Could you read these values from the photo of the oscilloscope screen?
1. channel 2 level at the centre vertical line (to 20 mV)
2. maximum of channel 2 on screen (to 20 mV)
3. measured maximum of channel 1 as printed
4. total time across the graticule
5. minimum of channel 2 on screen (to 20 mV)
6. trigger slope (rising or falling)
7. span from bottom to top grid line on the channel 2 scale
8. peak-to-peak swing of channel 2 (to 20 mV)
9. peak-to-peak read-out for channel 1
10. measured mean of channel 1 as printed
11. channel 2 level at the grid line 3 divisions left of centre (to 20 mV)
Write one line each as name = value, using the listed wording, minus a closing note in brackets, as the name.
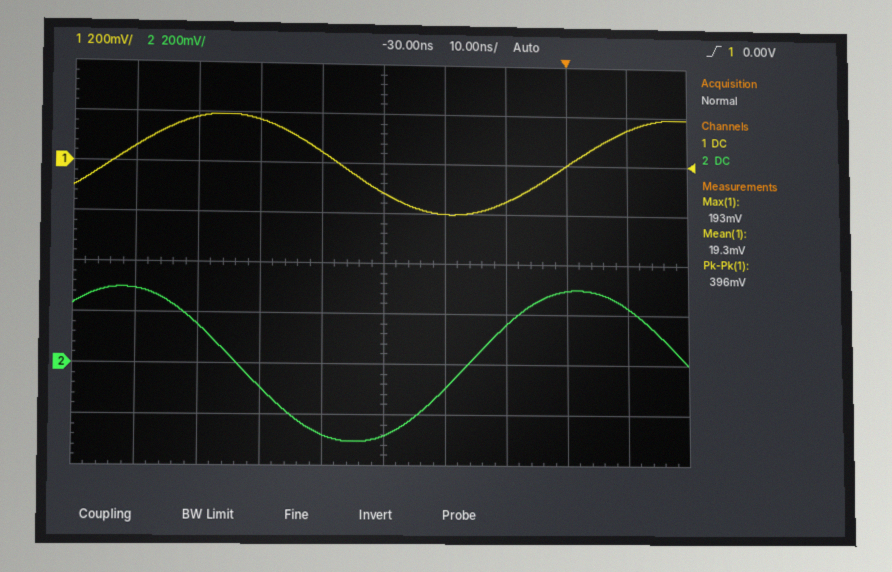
channel 2 level at the centre vertical line = -280 mV
maximum of channel 2 on screen = 300 mV
measured maximum of channel 1 as printed = 193 mV
total time across the graticule = 100 ns
minimum of channel 2 on screen = -300 mV
trigger slope = rising
span from bottom to top grid line on the channel 2 scale = 1.6 V
peak-to-peak swing of channel 2 = 600 mV
peak-to-peak read-out for channel 1 = 396 mV
measured mean of channel 1 as printed = 19.3 mV
channel 2 level at the grid line 3 divisions left of centre = 160 mV
